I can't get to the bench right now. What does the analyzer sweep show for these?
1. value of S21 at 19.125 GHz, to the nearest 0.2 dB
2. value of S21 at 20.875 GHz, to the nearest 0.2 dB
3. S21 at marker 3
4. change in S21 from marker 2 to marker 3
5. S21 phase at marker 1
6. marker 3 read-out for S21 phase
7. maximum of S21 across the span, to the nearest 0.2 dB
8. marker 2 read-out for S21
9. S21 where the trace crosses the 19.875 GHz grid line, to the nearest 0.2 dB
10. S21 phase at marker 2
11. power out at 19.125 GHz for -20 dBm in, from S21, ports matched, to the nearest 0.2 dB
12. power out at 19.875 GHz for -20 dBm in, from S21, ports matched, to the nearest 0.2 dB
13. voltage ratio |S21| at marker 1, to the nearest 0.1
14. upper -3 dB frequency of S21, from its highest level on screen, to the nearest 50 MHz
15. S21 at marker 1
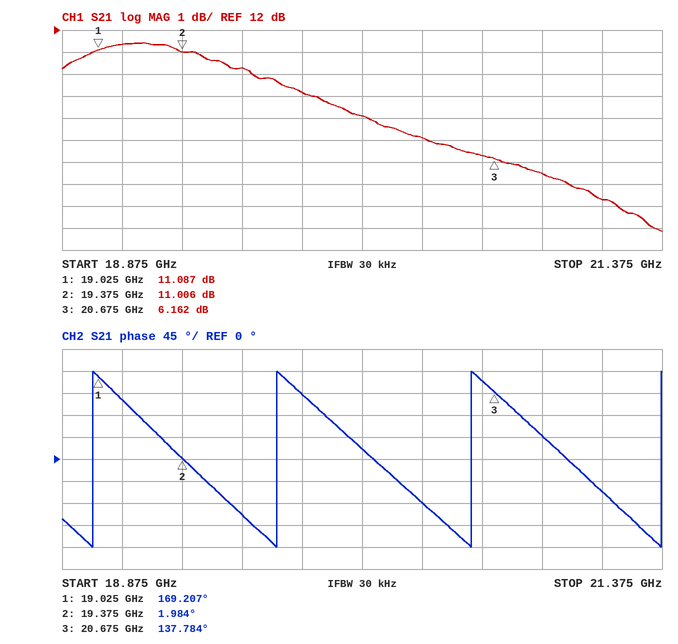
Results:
11.4 dB
5.4 dB
6.162 dB
-4.844 dB
169.207°
137.784°
11.4 dB
11.006 dB
9.2 dB
1.984°
-8.6 dBm
-10.8 dBm
3.6
20.05 GHz
11.087 dB
